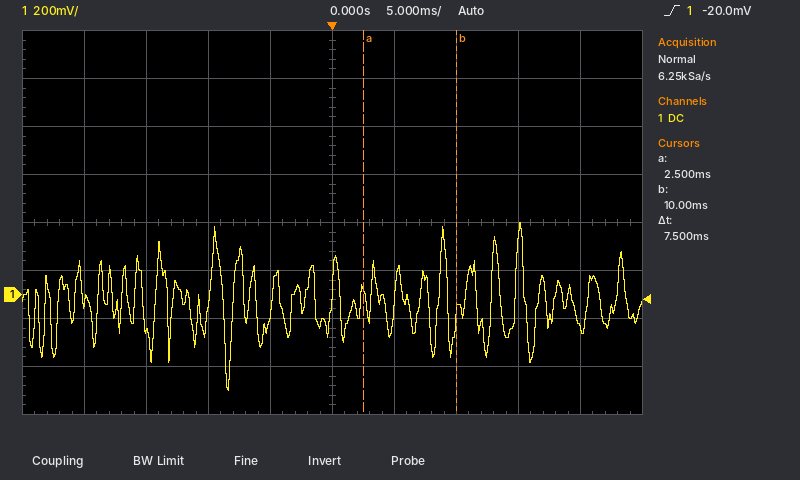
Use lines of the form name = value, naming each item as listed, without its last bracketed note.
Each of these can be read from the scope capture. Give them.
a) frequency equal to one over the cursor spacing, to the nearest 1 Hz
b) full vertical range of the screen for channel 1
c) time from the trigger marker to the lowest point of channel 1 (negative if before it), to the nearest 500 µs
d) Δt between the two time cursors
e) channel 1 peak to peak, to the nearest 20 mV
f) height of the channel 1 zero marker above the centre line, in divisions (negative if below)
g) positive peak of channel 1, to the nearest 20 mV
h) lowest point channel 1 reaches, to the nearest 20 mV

frequency equal to one over the cursor spacing, to the nearest 1 Hz = 133 Hz
full vertical range of the screen for channel 1 = 1.6 V
time from the trigger marker to the lowest point of channel 1 (negative if before it), to the nearest 500 µs = -8.5 ms
Δt between the two time cursors = 7.5 ms
channel 1 peak to peak, to the nearest 20 mV = 700 mV
height of the channel 1 zero marker above the centre line, in divisions = -1.5 div
positive peak of channel 1, to the nearest 20 mV = 300 mV
lowest point channel 1 reaches, to the nearest 20 mV = -400 mV
